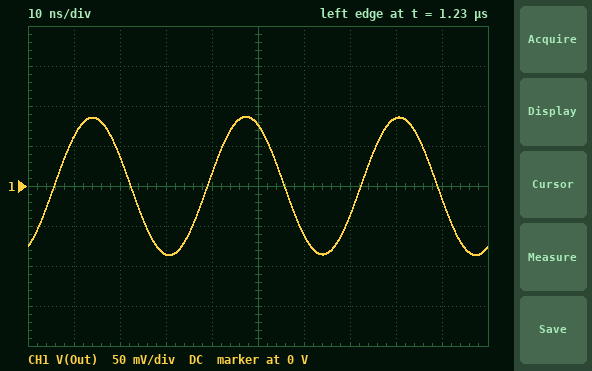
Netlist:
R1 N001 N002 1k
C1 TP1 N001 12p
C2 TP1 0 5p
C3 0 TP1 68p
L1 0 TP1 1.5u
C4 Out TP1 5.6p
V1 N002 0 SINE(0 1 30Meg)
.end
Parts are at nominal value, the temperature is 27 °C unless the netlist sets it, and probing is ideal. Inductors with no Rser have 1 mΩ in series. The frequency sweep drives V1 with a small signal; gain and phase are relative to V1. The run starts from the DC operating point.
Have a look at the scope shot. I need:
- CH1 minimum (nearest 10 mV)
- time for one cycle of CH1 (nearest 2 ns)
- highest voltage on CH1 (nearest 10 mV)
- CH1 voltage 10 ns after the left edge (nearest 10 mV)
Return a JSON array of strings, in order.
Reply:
["-90 mV", "34 ns", "90 mV", "60 mV"]
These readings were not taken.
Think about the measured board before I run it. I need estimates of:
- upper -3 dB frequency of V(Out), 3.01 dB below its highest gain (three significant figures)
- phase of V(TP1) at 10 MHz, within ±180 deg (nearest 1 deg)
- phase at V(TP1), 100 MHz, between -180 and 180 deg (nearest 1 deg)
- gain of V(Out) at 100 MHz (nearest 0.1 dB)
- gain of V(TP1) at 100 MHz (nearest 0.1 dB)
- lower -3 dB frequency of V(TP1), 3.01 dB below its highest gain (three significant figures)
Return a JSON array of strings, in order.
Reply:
["15.3 MHz", "139 deg", "-81 deg", "-33.1 dB", "-33.1 dB", "14.1 MHz"]
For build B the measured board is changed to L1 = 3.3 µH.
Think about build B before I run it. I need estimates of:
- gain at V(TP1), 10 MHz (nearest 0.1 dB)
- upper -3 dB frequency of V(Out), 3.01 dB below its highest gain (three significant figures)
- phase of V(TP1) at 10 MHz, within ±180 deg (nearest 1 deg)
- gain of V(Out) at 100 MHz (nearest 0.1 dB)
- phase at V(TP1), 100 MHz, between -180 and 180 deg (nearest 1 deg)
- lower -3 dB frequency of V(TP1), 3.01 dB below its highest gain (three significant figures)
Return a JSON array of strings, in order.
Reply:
["2.8 dB", "10.1 MHz", "19 deg", "-33.2 dB", "-81 deg", "9.40 MHz"]
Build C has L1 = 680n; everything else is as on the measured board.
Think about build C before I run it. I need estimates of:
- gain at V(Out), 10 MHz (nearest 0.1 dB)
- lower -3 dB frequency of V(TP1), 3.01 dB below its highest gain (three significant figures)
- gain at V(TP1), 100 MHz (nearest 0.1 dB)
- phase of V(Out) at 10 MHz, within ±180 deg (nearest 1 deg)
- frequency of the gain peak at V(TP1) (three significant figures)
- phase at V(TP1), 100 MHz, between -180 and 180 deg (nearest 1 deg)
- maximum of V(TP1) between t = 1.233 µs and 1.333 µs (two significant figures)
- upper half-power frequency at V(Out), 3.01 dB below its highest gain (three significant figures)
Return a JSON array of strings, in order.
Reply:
["-29.7 dB", "21.3 MHz", "-32.9 dB", "142 deg", "22.1 MHz", "-81 deg", "140 mV", "22.9 MHz"]
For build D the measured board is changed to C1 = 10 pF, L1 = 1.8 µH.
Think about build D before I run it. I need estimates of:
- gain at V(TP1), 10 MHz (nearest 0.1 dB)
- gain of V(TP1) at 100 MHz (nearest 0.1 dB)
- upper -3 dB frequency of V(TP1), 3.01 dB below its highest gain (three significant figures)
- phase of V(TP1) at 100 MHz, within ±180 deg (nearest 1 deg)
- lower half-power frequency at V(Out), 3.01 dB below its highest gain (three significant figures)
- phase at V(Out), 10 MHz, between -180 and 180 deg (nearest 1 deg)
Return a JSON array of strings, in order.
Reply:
["-17.1 dB", "-33.2 dB", "13.8 MHz", "-80 deg", "12.9 MHz", "144 deg"]
